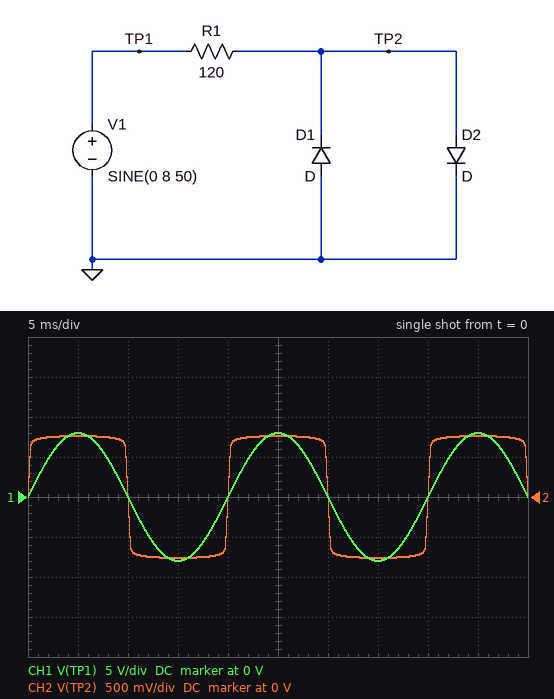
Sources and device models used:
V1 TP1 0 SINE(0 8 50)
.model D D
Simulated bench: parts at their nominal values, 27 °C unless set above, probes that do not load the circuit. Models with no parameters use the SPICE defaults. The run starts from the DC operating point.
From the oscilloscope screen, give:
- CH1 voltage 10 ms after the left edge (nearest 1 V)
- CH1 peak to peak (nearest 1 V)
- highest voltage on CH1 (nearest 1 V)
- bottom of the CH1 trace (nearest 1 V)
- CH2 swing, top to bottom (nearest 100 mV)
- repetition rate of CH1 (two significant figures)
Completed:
0 V
16 V
8 V
-8 V
1.5 V
50 Hz
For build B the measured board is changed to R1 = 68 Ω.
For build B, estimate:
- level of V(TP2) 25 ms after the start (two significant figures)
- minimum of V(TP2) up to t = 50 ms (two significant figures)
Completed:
780 mV
-780 mV
